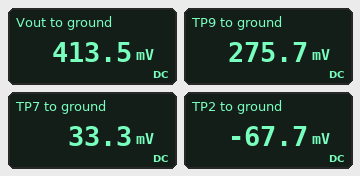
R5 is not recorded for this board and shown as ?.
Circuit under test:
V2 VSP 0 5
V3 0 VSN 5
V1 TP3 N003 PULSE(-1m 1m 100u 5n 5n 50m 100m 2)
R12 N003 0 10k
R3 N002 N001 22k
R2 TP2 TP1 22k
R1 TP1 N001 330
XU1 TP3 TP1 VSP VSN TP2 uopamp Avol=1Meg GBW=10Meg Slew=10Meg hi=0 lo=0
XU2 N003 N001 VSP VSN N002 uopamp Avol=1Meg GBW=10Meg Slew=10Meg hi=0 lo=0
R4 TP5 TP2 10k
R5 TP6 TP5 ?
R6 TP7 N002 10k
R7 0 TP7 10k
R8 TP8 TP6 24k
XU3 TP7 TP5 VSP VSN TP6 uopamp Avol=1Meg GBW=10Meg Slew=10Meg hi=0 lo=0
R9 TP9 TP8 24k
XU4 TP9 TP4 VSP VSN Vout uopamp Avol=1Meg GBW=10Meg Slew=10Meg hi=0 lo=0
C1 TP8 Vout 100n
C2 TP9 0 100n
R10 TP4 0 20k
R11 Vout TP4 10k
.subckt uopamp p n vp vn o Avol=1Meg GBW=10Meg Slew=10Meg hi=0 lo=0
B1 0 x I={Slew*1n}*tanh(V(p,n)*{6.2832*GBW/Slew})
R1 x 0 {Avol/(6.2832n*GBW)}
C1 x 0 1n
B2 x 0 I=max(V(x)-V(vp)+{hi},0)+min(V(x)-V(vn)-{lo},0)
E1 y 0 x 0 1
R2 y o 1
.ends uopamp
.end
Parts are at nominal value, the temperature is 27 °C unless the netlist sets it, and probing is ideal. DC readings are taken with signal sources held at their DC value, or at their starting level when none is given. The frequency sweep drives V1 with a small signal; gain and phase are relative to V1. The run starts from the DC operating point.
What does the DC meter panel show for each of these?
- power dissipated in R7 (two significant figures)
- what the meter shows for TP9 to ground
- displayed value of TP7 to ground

110 nW
275.7 mV
33.3 mV
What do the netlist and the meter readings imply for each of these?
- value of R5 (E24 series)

24 kΩ
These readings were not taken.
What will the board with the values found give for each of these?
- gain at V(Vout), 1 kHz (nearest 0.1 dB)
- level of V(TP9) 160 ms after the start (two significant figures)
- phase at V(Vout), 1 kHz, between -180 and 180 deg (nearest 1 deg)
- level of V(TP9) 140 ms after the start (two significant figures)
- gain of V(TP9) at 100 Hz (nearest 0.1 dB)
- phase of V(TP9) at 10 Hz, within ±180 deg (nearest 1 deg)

5.2 dB
290 mV
5 deg
-280 mV
40.5 dB
167 deg
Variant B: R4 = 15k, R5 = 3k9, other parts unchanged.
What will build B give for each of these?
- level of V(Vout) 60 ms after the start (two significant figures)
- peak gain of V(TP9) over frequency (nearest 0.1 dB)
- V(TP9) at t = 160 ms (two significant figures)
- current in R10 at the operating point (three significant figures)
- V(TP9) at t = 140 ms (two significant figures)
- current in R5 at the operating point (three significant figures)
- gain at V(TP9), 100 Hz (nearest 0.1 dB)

93 mV
35.5 dB
62 mV
2.98 µA
-60 mV
6.73 µA
27.2 dB
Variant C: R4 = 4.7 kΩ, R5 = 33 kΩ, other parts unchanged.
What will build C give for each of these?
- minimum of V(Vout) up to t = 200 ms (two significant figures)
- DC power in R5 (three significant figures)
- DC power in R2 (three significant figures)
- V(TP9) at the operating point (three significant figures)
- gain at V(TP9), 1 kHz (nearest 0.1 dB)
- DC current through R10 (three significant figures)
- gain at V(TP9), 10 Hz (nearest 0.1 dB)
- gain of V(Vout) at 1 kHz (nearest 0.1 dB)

-1.2 V
15.2 µW
202 nW
742 mV
10.3 dB
37.1 µA
57.4 dB
13.8 dB
